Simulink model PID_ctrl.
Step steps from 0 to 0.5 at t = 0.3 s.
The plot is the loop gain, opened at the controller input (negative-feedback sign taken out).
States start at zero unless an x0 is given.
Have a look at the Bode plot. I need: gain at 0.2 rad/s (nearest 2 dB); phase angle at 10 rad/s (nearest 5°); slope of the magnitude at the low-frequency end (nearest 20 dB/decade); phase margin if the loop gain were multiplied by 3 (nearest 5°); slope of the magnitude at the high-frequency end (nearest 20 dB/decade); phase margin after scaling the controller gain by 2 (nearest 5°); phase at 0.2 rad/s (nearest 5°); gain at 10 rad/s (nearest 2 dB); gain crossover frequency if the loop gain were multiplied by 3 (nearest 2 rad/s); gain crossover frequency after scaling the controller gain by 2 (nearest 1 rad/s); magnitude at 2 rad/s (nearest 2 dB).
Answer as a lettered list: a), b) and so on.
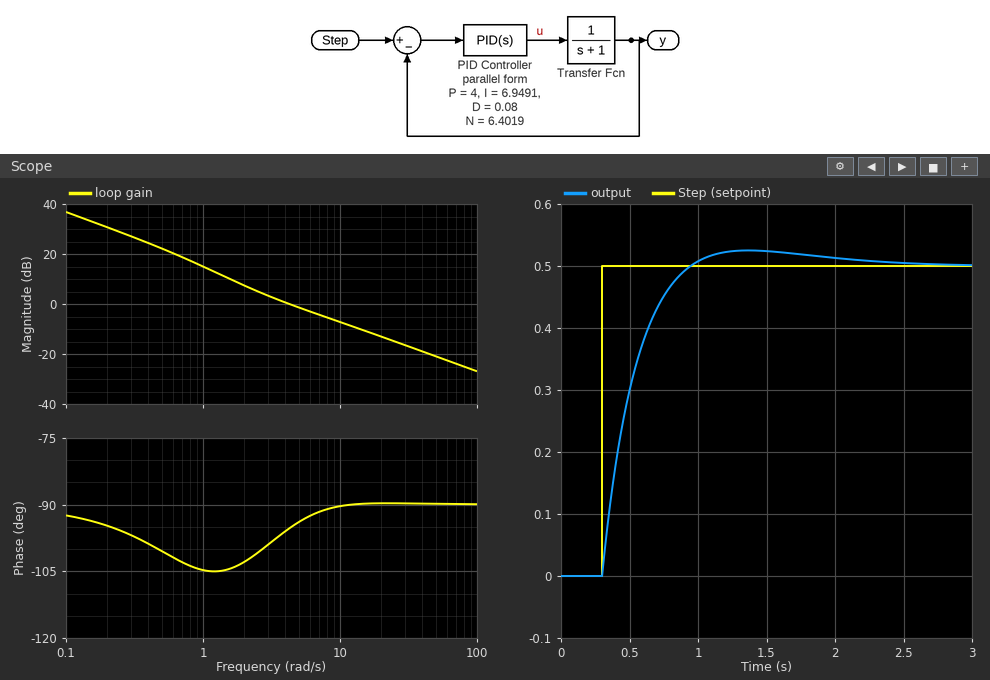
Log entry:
a) 30 dB
b) -90°
c) -20 dB/decade
d) 90°
e) -20 dB/decade
f) 90°
g) -95°
h) -8 dB
i) 14 rad/s
j) 9 rad/s
k) 8 dB
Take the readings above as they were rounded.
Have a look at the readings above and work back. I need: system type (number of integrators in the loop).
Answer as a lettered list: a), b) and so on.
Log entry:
a) 1
